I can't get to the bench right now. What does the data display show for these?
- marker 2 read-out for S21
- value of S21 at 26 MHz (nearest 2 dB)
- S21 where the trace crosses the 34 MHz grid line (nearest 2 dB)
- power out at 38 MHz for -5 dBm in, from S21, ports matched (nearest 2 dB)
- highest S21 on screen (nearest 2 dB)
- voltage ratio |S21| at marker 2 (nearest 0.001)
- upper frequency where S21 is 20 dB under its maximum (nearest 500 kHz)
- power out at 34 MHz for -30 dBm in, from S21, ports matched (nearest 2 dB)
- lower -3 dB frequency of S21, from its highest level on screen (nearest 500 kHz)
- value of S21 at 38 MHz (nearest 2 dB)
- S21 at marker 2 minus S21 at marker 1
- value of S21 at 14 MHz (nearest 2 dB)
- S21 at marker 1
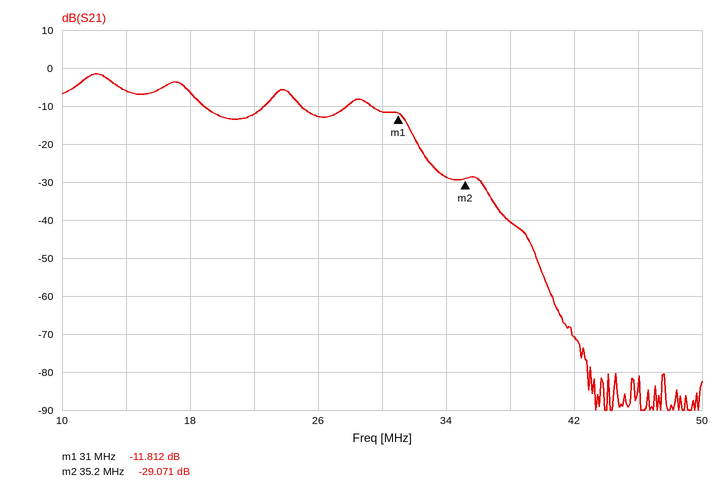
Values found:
-29.071 dB
-12 dB
-28 dB
-46 dBm
-2 dB
0.035
32.5 MHz
-58 dBm
11.0 MHz
-40 dB
-17.259 dB
-6 dB
-11.812 dB
